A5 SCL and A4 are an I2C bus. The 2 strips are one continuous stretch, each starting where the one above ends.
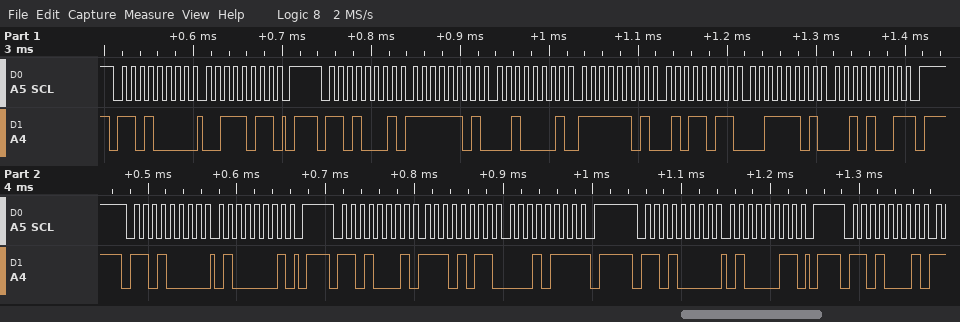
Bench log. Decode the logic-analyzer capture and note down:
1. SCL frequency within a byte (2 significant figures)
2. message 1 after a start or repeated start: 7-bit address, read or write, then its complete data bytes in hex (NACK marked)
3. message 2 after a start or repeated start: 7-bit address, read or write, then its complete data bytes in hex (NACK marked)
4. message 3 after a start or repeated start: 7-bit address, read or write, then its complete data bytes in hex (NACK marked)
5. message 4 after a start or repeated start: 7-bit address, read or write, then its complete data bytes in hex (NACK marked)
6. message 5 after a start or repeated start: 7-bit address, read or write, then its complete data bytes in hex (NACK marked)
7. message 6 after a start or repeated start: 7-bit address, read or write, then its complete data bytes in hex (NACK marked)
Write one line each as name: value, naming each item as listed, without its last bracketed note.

SCL frequency within a byte: 100 kHz
message 1 after a start or repeated start: 7-bit address, read or write, then its complete data bytes in hex: 0x68 write: 3B
message 2 after a start or repeated start: 7-bit address, read or write, then its complete data bytes in hex: 0x68 read: FD 21 FD 5B 3D 29 NACK
message 3 after a start or repeated start: 7-bit address, read or write, then its complete data bytes in hex: 0x68 write: 41
message 4 after a start or repeated start: 7-bit address, read or write, then its complete data bytes in hex: 0x68 read: EB 17 NACK
message 5 after a start or repeated start: 7-bit address, read or write, then its complete data bytes in hex: 0x68 write: 43
message 6 after a start or repeated start: 7-bit address, read or write, then its complete data bytes in hex: 0x68 read
